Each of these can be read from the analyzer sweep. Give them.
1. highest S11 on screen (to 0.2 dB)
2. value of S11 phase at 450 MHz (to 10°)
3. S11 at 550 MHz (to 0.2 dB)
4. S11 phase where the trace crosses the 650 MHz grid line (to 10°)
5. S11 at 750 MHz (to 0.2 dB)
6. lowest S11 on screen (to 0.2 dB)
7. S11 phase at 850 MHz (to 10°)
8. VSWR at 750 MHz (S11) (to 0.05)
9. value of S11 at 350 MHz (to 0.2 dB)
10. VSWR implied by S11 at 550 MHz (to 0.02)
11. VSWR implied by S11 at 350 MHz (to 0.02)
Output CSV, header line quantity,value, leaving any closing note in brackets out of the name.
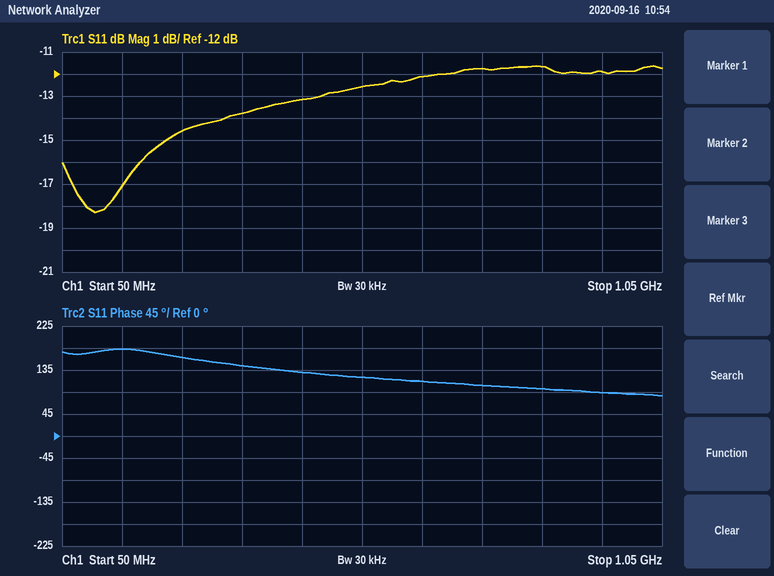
quantity,value
highest S11 on screen,-11.6 dB
value of S11 phase at 450 MHz,130°
S11 at 550 MHz,-12.6 dB
S11 phase where the trace crosses the 650 MHz grid line,110°
S11 at 750 MHz,-11.8 dB
lowest S11 on screen,-18.2 dB
S11 phase at 850 MHz,100°
VSWR at 750 MHz (S11),1.70
value of S11 at 350 MHz,-13.8 dB
VSWR implied by S11 at 550 MHz,1.62
VSWR implied by S11 at 350 MHz,1.52
